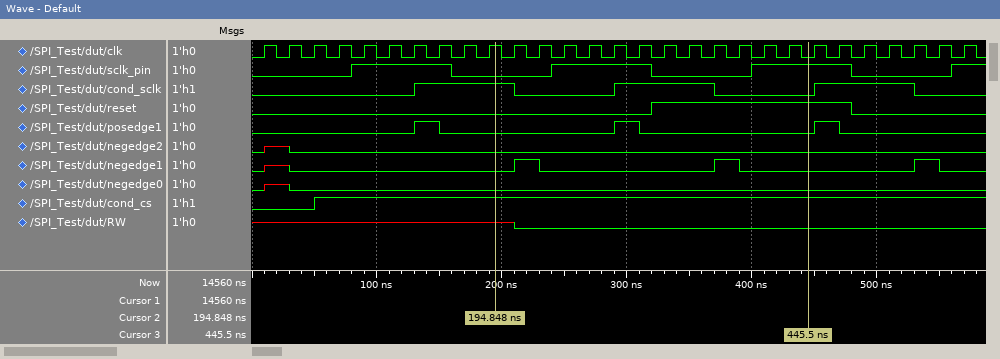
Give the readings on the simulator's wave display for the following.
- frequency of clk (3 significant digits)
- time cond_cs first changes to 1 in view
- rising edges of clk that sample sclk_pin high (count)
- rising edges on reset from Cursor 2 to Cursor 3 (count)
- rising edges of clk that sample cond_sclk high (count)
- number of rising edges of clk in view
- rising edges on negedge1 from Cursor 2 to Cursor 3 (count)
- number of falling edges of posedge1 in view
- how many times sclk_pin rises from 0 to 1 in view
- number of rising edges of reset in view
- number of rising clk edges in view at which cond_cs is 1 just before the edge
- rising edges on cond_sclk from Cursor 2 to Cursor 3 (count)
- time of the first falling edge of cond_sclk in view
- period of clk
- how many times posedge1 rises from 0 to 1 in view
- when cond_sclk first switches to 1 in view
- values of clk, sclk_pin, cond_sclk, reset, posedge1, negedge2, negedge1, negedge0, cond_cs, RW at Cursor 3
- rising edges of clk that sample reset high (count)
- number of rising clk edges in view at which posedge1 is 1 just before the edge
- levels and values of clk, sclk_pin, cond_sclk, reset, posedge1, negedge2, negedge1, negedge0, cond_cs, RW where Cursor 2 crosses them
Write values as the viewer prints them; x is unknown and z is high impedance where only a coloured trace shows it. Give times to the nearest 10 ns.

50.0 MHz
50 ns
13
1
12
29
2
3
4
1
26
1
210 ns
20 ns
3
130 ns
clk=0, sclk_pin=1, cond_sclk=0, reset=1, posedge1=0, negedge2=0, negedge1=0, negedge0=0, cond_cs=1, RW=0
8
3
clk=1, sclk_pin=0, cond_sclk=1, reset=0, posedge1=0, negedge2=0, negedge1=0, negedge0=0, cond_cs=1, RW=x
